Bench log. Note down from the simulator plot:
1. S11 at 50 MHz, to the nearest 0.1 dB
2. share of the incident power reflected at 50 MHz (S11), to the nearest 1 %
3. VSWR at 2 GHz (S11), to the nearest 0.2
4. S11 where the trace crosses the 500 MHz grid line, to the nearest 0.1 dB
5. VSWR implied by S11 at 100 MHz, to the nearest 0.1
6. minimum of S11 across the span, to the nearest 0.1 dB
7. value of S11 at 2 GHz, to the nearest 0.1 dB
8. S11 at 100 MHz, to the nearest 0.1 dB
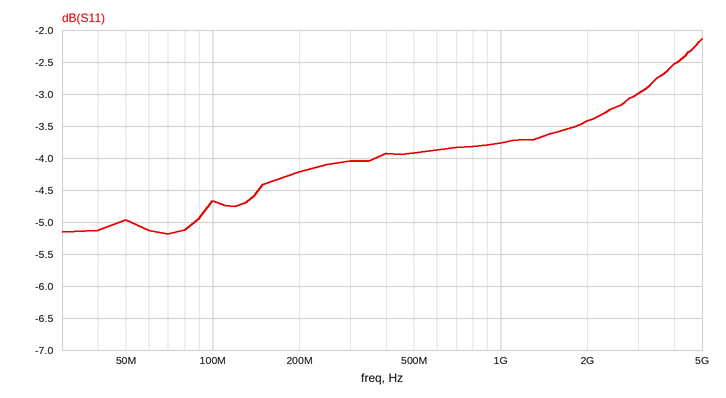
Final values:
-5.0 dB
32 %
5.2
-3.9 dB
3.8
-5.2 dB
-3.4 dB
-4.7 dB
